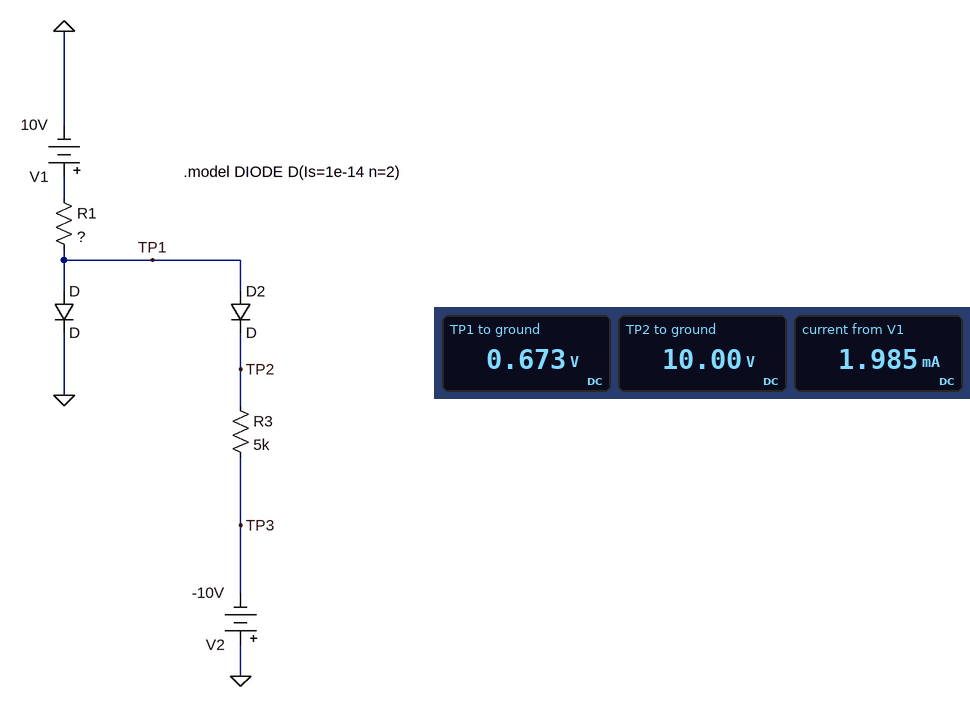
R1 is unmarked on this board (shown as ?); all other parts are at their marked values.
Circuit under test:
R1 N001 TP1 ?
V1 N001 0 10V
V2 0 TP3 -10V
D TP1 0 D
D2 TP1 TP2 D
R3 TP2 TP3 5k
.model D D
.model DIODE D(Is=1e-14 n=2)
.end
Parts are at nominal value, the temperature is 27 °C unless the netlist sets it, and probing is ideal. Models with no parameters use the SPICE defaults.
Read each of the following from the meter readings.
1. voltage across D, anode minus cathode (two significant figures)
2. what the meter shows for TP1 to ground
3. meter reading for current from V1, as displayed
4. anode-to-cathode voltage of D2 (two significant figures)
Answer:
670 mV
0.673 V
1.985 mA
-9.3 V
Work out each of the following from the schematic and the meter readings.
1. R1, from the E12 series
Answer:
4.7 kΩ
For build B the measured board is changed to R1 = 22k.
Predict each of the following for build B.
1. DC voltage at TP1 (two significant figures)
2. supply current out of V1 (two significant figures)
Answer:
630 mV
430 µA
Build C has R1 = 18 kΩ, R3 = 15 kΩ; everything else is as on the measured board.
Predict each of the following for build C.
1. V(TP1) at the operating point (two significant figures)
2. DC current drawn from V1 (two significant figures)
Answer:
640 mV
520 µA
